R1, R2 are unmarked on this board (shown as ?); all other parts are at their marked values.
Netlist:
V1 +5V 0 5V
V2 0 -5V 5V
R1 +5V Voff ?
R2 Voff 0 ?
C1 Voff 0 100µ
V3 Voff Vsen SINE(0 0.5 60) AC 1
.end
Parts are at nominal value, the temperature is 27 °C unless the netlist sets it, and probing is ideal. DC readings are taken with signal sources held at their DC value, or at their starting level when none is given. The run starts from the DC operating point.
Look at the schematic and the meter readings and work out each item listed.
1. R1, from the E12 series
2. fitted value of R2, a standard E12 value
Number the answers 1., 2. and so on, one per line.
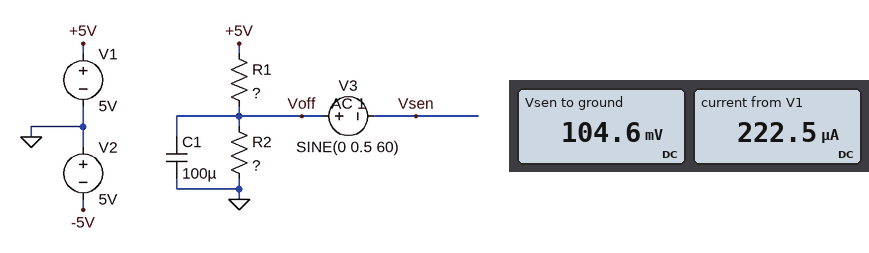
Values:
1. 22 kΩ
2. 470 Ω
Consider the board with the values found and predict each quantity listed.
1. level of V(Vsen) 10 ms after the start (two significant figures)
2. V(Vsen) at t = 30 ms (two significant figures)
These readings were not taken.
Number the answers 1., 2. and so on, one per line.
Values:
1. 400 mV
2. 580 mV
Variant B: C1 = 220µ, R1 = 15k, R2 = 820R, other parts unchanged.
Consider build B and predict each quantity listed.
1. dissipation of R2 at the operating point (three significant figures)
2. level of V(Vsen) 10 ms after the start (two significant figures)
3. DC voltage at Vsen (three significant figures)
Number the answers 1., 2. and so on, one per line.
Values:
1. 81.9 µW
2. 550 mV
3. 259 mV
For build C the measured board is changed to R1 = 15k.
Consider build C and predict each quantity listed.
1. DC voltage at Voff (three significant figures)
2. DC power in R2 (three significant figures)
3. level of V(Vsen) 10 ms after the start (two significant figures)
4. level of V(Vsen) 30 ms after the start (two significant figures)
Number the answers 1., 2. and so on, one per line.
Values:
1. 152 mV
2. 49.1 µW
3. 450 mV
4. 630 mV
